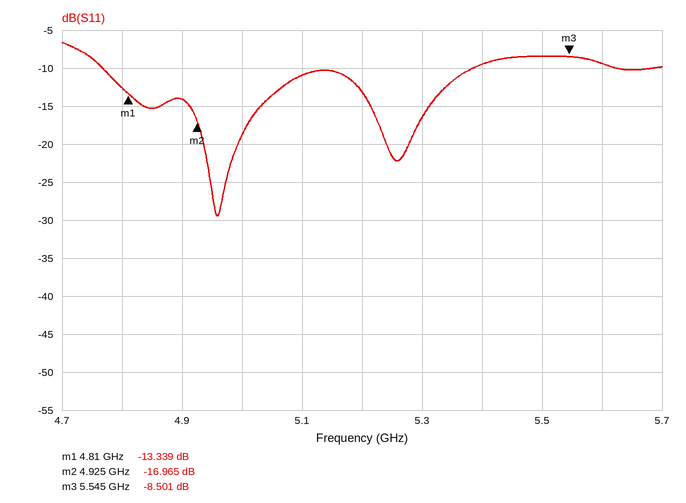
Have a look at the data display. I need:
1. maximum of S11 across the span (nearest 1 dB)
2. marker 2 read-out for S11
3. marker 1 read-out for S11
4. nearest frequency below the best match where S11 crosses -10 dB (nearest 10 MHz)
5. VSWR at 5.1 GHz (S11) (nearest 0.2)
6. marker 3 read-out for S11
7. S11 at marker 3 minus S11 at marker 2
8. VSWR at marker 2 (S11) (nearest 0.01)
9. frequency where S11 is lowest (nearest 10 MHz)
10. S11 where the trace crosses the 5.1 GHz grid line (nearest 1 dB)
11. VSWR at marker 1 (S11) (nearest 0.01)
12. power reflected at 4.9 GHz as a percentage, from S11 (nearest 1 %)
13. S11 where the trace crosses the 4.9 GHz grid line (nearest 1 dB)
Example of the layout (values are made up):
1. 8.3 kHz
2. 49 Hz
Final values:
1. -7 dB
2. -16.965 dB
3. -13.339 dB
4. 4.77 GHz
5. 1.8
6. -8.501 dB
7. 8.464 dB
8. 1.33
9. 4.96 GHz
10. -11 dB
11. 1.55
12. 4 %
13. -14 dB
